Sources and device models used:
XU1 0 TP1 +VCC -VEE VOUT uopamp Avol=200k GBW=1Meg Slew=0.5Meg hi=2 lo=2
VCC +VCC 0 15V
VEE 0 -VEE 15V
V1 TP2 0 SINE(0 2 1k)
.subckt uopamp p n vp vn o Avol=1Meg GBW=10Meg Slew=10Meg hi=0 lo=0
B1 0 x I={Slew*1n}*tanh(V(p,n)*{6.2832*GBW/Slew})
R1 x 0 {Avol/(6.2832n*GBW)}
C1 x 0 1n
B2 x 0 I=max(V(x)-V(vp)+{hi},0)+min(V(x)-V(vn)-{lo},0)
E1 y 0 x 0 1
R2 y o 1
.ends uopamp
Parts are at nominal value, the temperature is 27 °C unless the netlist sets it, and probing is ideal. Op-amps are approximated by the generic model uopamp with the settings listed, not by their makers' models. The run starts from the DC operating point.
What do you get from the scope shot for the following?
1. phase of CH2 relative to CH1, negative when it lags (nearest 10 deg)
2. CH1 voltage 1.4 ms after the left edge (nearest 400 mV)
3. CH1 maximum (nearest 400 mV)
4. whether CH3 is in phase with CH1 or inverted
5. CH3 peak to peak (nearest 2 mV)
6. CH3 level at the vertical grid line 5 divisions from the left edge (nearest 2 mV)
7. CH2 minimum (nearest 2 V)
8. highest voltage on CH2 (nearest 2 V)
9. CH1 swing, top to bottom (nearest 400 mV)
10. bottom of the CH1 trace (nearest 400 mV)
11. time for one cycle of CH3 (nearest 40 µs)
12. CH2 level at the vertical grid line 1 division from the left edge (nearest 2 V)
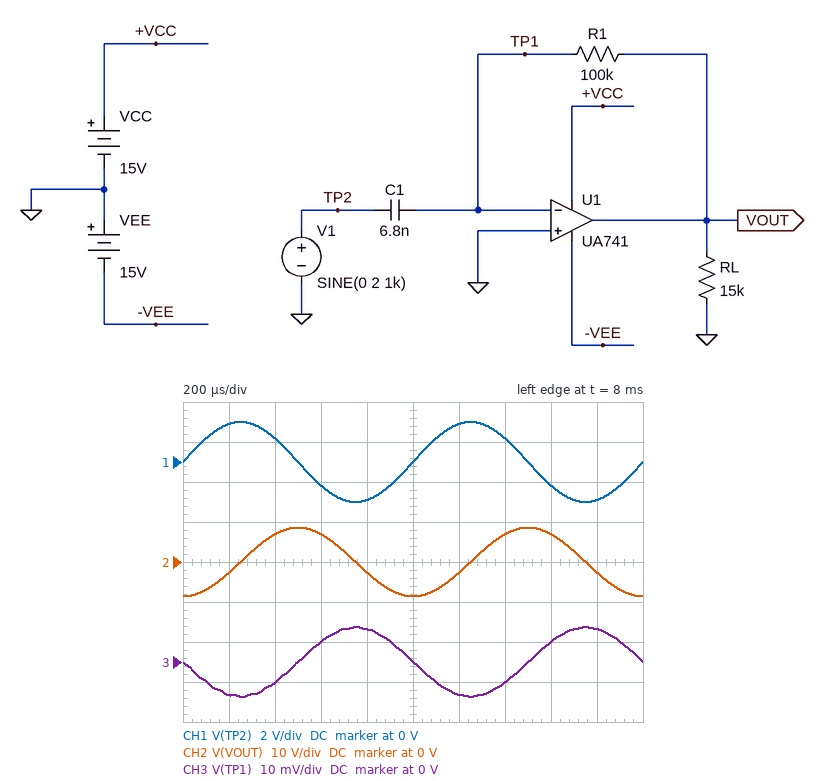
-90 deg
1.2 V
2.0 V
inverted
18 mV
0 V
-8 V
8 V
4.0 V
-2.0 V
1.00 ms
-2 V
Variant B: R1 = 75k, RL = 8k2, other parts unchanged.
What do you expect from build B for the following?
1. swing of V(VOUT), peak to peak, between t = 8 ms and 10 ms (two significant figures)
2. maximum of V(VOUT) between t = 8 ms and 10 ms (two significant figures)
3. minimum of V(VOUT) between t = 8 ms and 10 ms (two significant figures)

13 V
6.4 V
-6.4 V
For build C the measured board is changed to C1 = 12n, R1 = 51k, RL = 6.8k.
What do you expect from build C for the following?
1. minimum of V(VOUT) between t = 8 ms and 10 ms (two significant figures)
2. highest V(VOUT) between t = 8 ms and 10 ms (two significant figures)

-7.7 V
7.7 V
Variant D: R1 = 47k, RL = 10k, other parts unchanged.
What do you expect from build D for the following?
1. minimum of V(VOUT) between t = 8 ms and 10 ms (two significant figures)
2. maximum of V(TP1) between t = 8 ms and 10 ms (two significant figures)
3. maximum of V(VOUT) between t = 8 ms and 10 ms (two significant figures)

-4.0 V
4.0 mV
4.0 V
